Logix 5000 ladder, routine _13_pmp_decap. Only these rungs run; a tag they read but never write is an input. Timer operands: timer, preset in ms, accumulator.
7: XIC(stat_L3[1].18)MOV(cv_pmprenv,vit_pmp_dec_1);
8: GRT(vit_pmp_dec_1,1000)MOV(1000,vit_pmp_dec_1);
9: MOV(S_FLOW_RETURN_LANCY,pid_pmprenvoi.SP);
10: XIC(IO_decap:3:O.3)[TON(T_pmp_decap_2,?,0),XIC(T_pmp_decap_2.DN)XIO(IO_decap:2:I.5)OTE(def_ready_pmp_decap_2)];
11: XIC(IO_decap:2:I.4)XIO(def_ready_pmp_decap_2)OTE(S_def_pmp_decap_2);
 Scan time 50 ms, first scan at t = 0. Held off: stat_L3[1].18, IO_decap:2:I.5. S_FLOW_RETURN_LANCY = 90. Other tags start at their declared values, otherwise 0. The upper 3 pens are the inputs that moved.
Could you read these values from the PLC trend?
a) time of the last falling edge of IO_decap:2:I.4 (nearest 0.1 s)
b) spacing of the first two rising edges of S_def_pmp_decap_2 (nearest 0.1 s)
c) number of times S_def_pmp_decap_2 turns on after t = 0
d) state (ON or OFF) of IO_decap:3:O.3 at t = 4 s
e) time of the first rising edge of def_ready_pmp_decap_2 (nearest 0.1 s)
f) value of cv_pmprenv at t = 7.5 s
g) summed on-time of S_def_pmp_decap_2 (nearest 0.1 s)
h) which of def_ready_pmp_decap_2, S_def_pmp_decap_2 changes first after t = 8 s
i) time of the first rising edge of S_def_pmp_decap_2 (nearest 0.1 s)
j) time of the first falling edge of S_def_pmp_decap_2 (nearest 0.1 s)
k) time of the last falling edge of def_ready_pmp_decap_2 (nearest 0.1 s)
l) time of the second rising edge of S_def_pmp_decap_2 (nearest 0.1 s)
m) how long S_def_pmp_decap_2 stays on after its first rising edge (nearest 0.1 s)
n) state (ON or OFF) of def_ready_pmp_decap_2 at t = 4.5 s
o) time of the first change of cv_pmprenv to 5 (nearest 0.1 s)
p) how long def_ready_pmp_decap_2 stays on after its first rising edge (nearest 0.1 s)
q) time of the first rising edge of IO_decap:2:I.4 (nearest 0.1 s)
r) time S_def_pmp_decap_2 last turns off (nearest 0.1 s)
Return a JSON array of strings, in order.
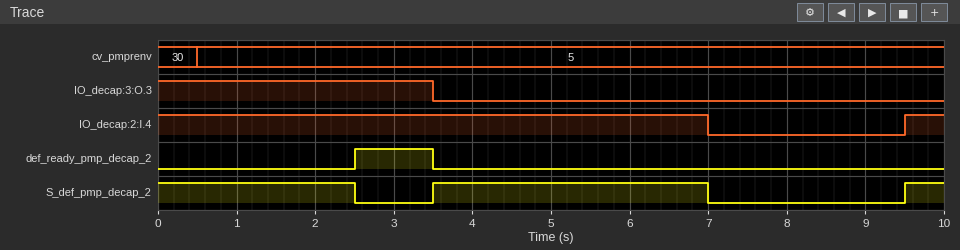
["7.0 s", "6.0 s", "2", "OFF", "2.5 s", "5", "6.5 s", "S_def_pmp_decap_2", "3.5 s", "2.5 s", "3.5 s", "9.5 s", "3.5 s", "OFF", "0.5 s", "1.0 s", "9.5 s", "7.0 s"]
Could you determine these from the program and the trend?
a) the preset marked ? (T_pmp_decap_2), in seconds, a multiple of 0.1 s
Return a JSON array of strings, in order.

["2.5 s"]
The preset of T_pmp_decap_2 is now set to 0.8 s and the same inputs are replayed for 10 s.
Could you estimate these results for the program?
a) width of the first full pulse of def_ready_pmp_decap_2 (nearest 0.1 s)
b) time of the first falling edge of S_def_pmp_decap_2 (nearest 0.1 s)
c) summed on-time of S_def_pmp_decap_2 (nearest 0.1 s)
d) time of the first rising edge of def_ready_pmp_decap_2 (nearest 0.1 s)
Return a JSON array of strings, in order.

["2.7 s", "0.8 s", "4.8 s", "0.8 s"]
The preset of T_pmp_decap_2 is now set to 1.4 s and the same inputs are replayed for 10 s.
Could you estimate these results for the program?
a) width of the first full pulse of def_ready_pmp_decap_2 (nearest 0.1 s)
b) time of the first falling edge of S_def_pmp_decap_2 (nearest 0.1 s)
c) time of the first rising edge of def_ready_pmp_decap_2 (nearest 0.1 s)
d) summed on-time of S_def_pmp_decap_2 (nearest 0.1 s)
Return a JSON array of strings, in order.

["2.1 s", "1.4 s", "1.4 s", "5.4 s"]
